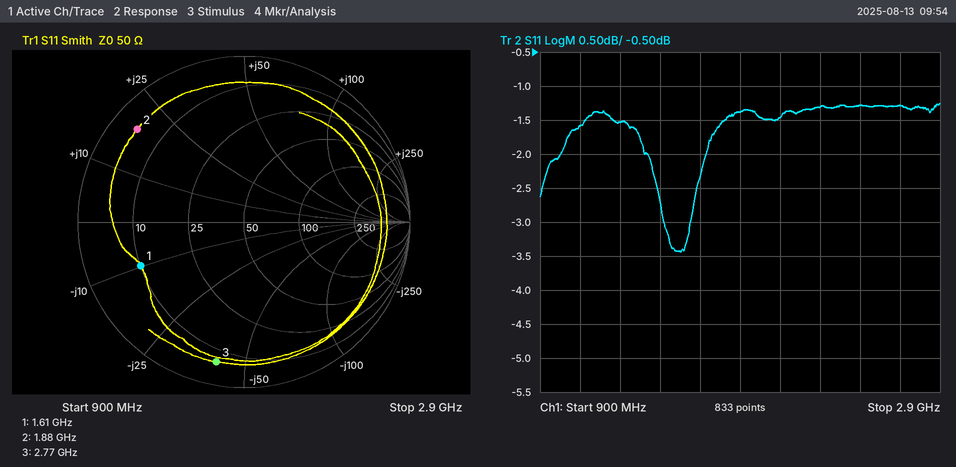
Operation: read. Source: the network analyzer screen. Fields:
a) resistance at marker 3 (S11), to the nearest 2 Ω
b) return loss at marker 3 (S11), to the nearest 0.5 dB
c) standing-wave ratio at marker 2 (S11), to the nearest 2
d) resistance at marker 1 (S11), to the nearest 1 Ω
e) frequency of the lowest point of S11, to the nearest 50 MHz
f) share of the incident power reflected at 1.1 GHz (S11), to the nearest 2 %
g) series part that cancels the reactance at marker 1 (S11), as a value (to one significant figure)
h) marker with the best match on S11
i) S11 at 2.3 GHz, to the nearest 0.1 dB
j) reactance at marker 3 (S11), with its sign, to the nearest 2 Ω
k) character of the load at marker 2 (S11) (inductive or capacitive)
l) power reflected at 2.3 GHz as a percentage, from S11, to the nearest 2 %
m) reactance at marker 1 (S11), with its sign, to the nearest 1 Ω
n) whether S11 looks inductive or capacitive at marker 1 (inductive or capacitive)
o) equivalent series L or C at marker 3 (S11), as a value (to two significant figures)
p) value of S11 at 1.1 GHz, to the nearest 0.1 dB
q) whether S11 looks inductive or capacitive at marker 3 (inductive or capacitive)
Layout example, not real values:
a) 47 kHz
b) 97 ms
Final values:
a) 6 Ω
b) 1.5 dB
c) 12
d) 10 Ω
e) 1.60 GHz
f) 70 %
g) 1.0 nH
h) marker 1
i) -1.3 dB
j) -40 Ω
k) inductive
l) 74 %
m) -10 Ω
n) capacitive
o) 1.4 pF
p) -1.6 dB
q) capacitive
